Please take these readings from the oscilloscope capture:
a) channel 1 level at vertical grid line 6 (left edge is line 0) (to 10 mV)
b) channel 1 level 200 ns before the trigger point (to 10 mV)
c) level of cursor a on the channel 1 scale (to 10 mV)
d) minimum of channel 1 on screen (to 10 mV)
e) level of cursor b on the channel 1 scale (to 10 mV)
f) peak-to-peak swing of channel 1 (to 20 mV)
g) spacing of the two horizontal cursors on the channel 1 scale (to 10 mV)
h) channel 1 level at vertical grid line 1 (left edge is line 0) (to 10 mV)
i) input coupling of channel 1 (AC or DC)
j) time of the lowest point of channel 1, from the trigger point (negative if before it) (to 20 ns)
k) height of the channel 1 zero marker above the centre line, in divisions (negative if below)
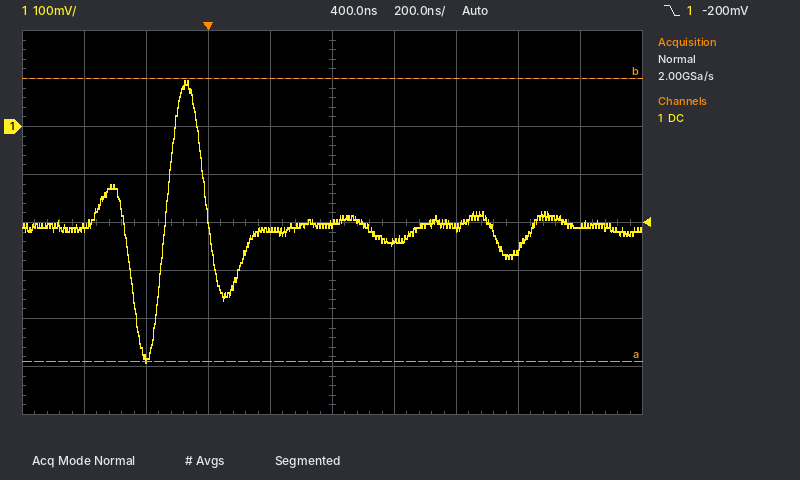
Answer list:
-240 mV
-480 mV
-490 mV
-490 mV
100 mV
580 mV
590 mV
-210 mV
DC
-200 ns
+2.0 div
